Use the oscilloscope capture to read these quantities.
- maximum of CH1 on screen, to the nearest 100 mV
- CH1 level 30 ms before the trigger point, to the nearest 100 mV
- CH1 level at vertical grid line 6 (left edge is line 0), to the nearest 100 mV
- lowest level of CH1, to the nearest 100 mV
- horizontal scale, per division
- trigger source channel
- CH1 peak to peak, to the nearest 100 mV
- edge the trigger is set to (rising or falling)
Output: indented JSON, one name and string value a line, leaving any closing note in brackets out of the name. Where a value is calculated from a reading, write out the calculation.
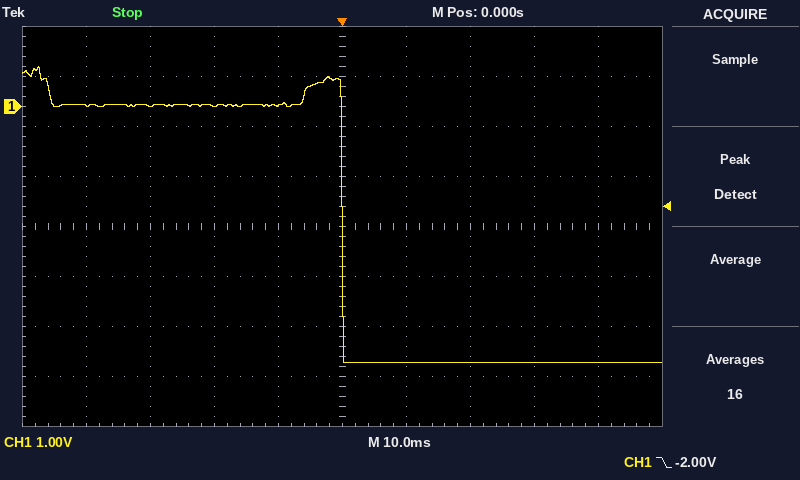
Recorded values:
{
  "maximum of CH1 on screen, to the nearest 100 mV": "800 mV",
  "CH1 level 30 ms before the trigger point, to the nearest 100 mV": "0.0 V",
  "CH1 level at vertical grid line 6 (left edge is line 0), to the nearest 100 mV": "-5.1 V",
  "lowest level of CH1, to the nearest 100 mV": "-5.1 V",
  "horizontal scale, per division": "10 ms",
  "trigger source channel": "CH1",
  "CH1 peak to peak, to the nearest 100 mV": "800 mV − (-5.1 V) = 5.9 V",
  "edge the trigger is set to": "falling"
}
